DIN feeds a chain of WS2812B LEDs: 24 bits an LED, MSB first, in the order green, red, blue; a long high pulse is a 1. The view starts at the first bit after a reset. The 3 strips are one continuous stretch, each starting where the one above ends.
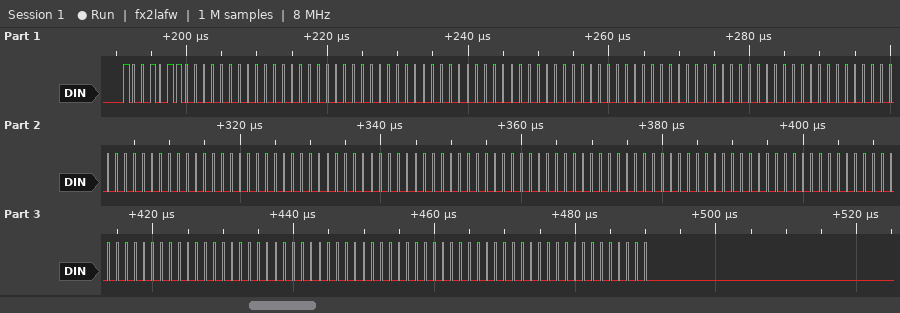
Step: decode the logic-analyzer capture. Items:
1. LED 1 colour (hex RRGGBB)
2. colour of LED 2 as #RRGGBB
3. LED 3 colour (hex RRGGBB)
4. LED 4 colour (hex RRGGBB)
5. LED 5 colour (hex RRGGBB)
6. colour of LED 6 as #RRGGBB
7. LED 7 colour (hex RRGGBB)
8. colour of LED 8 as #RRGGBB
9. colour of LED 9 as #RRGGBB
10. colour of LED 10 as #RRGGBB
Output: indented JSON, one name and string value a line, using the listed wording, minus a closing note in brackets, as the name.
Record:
{
  "LED 1 colour": "#009600",
  "colour of LED 2 as #RRGGBB": "#000000",
  "LED 3 colour": "#000000",
  "LED 4 colour": "#000000",
  "LED 5 colour": "#000000",
  "colour of LED 6 as #RRGGBB": "#000000",
  "LED 7 colour": "#000000",
  "colour of LED 8 as #RRGGBB": "#000000",
  "colour of LED 9 as #RRGGBB": "#000000",
  "colour of LED 10 as #RRGGBB": "#000000"
}
